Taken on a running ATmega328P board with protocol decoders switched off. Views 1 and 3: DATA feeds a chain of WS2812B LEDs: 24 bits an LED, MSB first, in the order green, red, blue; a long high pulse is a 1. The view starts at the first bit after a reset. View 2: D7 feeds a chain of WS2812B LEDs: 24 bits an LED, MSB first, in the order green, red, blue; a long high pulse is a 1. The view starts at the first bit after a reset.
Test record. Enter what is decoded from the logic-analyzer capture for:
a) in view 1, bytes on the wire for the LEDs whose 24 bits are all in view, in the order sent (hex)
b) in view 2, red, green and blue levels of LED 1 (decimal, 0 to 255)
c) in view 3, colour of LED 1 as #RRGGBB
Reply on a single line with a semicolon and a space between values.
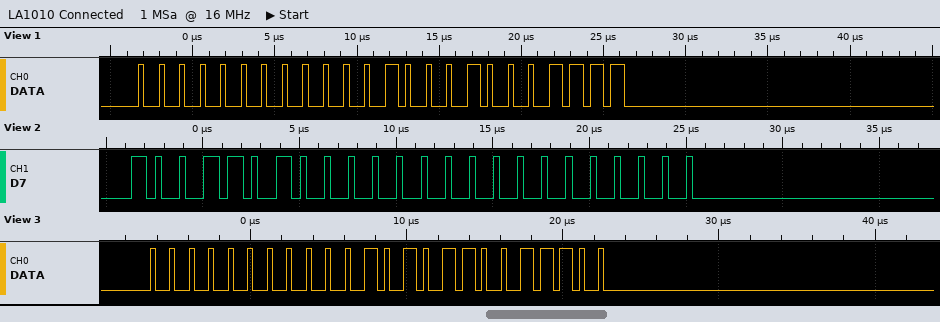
00 08 8F; 0, 154, 0; #15009C
